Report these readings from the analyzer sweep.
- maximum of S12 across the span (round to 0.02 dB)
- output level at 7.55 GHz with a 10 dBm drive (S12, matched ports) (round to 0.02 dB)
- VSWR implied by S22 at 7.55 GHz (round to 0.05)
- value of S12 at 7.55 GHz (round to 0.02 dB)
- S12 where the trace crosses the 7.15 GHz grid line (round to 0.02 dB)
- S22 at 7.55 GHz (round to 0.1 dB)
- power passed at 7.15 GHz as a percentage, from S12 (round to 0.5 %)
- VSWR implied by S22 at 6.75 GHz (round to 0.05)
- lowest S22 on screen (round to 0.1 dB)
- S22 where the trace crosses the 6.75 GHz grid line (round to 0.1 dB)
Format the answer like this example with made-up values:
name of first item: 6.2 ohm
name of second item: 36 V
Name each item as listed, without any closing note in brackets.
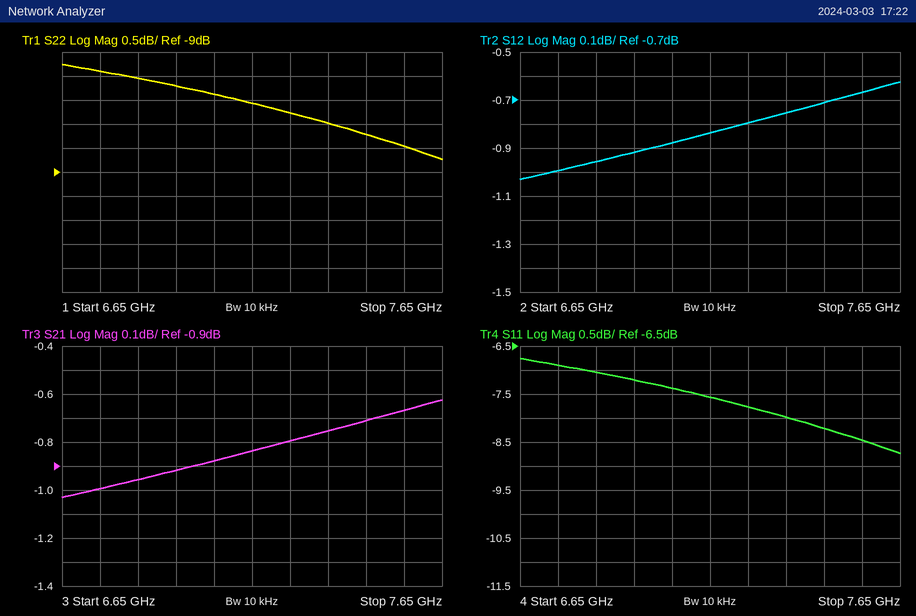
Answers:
maximum of S12 across the span: -0.62 dB
output level at 7.55 GHz with a 10 dBm drive (S12, matched ports): 9.34 dBm
VSWR implied by S22 at 7.55 GHz: 2.20
value of S12 at 7.55 GHz: -0.66 dB
S12 where the trace crosses the 7.15 GHz grid line: -0.84 dB
S22 at 7.55 GHz: -8.5 dB
power passed at 7.15 GHz as a percentage, from S12: 82.5 %
VSWR implied by S22 at 6.75 GHz: 2.65
lowest S22 on screen: -8.7 dB
S22 where the trace crosses the 6.75 GHz grid line: -6.9 dB
